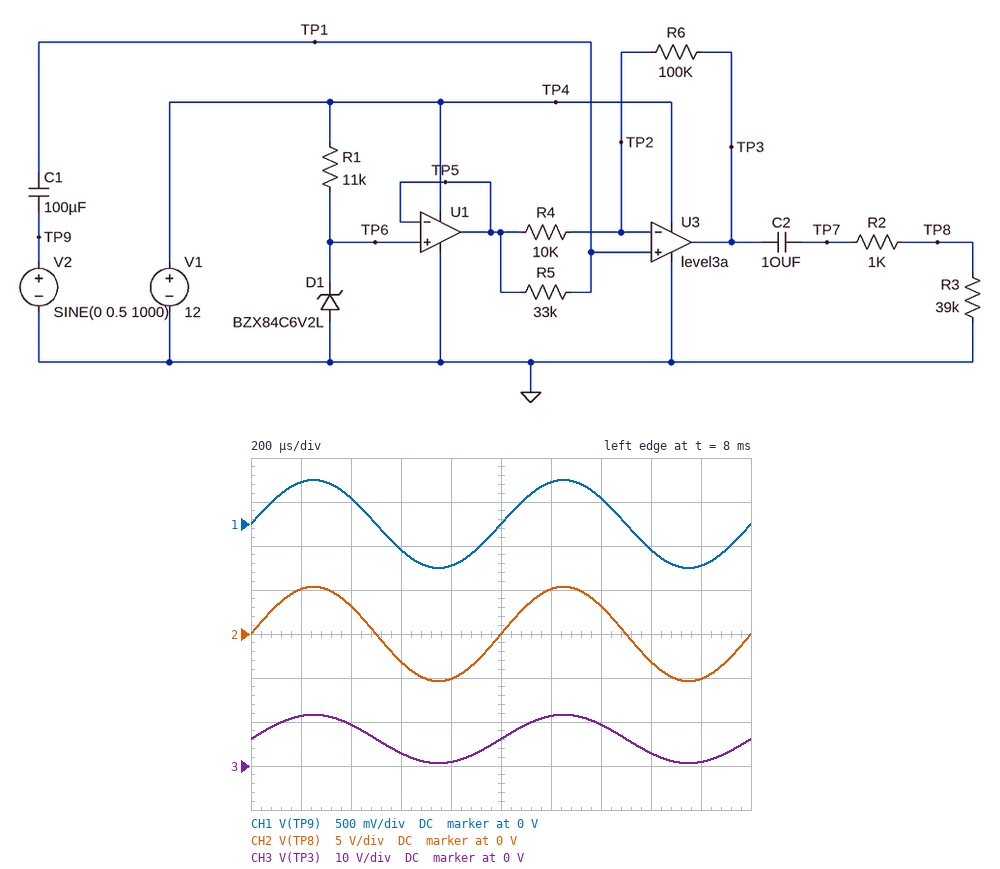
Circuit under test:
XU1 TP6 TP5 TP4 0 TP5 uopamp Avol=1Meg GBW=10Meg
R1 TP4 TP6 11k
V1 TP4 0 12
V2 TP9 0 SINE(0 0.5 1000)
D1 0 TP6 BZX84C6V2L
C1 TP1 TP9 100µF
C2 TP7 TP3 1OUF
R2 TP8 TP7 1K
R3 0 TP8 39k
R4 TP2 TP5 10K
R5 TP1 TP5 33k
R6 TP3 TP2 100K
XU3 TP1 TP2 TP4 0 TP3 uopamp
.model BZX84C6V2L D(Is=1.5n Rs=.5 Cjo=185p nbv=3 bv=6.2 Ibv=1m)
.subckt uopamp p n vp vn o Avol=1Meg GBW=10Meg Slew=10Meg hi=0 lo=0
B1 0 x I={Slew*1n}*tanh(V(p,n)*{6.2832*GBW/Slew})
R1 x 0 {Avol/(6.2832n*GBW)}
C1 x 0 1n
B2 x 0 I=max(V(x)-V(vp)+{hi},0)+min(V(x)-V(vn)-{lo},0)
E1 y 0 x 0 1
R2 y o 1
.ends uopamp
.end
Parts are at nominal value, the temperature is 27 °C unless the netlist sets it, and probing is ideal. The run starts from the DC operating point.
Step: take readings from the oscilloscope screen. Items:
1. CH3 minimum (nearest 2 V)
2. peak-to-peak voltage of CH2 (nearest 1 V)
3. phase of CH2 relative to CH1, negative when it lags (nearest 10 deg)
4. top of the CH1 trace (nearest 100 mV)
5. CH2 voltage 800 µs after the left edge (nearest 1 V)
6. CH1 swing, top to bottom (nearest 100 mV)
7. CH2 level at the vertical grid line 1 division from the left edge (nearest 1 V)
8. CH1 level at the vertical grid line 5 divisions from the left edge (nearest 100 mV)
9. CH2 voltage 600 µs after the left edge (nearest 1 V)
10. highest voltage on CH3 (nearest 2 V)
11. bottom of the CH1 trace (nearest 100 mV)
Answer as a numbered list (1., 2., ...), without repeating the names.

1. 0 V
2. 11 V
3. 0 deg
4. 500 mV
5. -5 V
6. 1.0 V
7. 5 V
8. 0 V
9. -3 V
10. 12 V
11. -500 mV
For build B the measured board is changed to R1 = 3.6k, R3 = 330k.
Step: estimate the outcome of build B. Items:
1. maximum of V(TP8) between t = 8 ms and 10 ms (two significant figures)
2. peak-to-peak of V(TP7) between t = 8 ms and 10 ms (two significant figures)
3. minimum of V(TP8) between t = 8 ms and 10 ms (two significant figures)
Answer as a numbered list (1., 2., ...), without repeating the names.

1. 5.5 V
2. 11 V
3. -5.5 V
